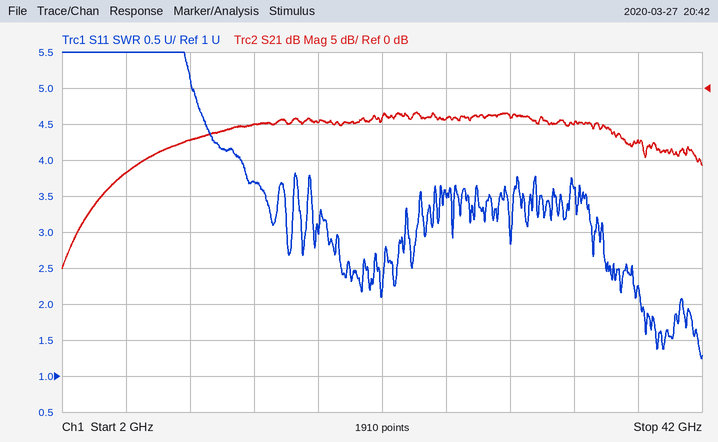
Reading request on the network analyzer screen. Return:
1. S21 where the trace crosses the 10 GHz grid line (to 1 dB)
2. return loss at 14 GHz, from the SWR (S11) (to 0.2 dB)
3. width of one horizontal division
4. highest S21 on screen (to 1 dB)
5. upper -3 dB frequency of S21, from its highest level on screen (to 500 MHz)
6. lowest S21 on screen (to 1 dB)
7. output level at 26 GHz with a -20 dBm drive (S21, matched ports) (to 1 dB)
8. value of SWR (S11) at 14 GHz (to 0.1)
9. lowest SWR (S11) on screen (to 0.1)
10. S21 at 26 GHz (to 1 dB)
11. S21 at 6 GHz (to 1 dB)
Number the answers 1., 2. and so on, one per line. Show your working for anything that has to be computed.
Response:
1. -7 dB
2. −20 log10((3.7 − 1)/(3.7 + 1)) ≈ 4.8 dB
3. 4 GHz
4. -3 dB
5. 36.5 GHz
6. -25 dB
7. -20 dBm + (-4 dB) = -24 dBm
8. 3.7
9. 1.2
10. -4 dB
11. -12 dB
